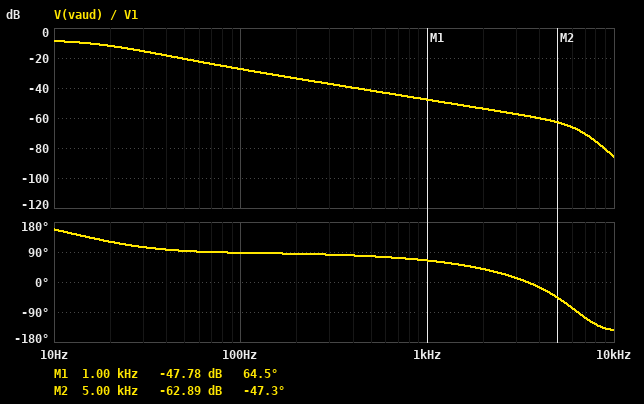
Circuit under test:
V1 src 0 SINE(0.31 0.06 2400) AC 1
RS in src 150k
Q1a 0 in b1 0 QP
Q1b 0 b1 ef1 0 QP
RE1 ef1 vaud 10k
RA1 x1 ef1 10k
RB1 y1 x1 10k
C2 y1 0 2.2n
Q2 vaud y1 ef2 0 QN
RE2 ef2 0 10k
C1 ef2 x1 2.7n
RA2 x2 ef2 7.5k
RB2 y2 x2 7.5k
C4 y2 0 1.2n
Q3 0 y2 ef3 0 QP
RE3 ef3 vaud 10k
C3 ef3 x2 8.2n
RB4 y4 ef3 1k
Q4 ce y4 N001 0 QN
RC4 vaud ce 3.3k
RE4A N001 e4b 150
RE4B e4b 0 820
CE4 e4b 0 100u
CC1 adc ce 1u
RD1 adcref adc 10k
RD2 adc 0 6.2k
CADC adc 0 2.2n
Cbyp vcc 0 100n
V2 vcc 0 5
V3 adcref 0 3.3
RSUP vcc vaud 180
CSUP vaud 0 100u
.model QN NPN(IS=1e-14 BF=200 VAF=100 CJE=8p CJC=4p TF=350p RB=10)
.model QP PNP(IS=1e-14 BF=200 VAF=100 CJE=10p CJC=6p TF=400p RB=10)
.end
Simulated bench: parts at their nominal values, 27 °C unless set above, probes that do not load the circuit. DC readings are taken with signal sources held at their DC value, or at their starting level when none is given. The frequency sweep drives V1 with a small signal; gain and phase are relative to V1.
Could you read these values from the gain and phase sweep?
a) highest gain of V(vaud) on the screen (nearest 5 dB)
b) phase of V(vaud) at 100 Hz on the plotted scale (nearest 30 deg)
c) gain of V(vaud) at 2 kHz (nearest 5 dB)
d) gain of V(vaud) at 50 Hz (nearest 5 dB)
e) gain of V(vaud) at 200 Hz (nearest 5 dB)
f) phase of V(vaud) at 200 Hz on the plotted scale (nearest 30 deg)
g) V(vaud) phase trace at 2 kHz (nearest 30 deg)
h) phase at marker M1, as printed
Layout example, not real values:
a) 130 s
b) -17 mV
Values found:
a) -10 dB
b) 90 deg
c) -55 dB
d) -20 dB
e) -35 dB
f) 90 deg
g) 30 deg
h) 64.5 deg
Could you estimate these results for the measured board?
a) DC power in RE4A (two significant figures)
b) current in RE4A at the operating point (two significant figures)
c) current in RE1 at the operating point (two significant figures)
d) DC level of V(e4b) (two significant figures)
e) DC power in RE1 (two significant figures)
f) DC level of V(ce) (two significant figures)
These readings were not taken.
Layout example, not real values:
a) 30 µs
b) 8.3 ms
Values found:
a) 110 µW
b) 850 µA
c) 330 µA
d) 700 mV
e) 1.1 mW
f) 1.9 V
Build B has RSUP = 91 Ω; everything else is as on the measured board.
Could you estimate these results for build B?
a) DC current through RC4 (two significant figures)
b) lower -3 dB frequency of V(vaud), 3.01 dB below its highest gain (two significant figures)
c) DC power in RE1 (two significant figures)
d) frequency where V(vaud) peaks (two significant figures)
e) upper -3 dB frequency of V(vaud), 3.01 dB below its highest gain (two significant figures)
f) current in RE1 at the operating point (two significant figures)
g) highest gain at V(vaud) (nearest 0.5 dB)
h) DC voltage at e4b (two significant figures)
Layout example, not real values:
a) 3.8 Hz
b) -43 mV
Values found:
a) 850 µA
b) 4.5 Hz
c) 1.2 mW
d) 11 Hz
e) 26 Hz
f) 340 µA
g) -12.0 dB
h) 700 mV
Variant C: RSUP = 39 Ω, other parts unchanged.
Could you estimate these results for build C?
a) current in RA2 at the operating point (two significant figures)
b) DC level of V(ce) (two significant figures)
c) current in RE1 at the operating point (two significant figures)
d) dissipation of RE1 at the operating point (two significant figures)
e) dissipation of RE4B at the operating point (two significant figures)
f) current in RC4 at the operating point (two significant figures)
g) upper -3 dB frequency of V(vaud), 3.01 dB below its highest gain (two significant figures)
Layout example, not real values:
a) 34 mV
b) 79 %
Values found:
a) 1.7 µA
b) 2.1 V
c) 350 µA
d) 1.2 mW
e) 600 µW
f) 850 µA
g) 38 Hz
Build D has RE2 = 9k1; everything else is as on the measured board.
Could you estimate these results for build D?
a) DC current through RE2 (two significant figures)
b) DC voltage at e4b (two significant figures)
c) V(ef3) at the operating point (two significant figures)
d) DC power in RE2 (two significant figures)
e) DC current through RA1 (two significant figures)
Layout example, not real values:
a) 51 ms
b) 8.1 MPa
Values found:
a) 91 µA
b) 690 mV
c) 1.5 V
d) 75 µW
e) 430 nA
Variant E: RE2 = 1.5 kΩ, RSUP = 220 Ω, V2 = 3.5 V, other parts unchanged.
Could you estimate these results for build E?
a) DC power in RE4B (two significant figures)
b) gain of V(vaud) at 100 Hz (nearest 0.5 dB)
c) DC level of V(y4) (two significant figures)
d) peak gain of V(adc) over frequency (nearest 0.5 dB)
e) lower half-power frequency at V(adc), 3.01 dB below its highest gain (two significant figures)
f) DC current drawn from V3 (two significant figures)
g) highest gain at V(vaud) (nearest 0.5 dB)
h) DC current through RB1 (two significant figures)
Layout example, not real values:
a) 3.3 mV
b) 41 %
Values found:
a) 410 µW
b) -30.5 dB
c) 1.3 V
d) 13.5 dB
e) 31 Hz
f) 200 µA
g) -11.0 dB
h) 2.3 µA
